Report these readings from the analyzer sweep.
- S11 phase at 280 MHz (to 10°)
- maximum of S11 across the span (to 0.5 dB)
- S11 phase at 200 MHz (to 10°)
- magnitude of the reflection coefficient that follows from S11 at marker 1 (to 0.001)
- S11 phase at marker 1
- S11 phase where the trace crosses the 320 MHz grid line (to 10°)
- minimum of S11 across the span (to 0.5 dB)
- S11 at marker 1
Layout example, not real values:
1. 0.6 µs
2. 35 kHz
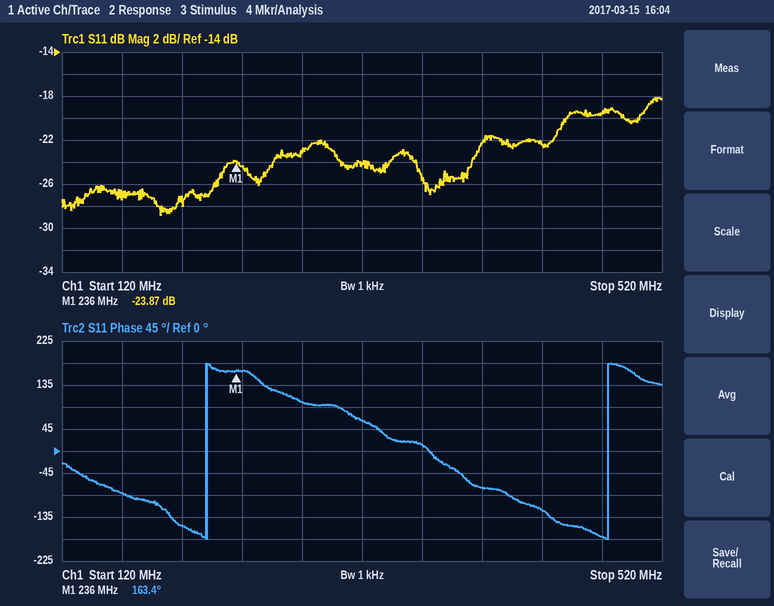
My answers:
1. 100°
2. -18.0 dB
3. -150°
4. 0.064
5. 163.4°
6. 60°
7. -29.0 dB
8. -23.87 dB
